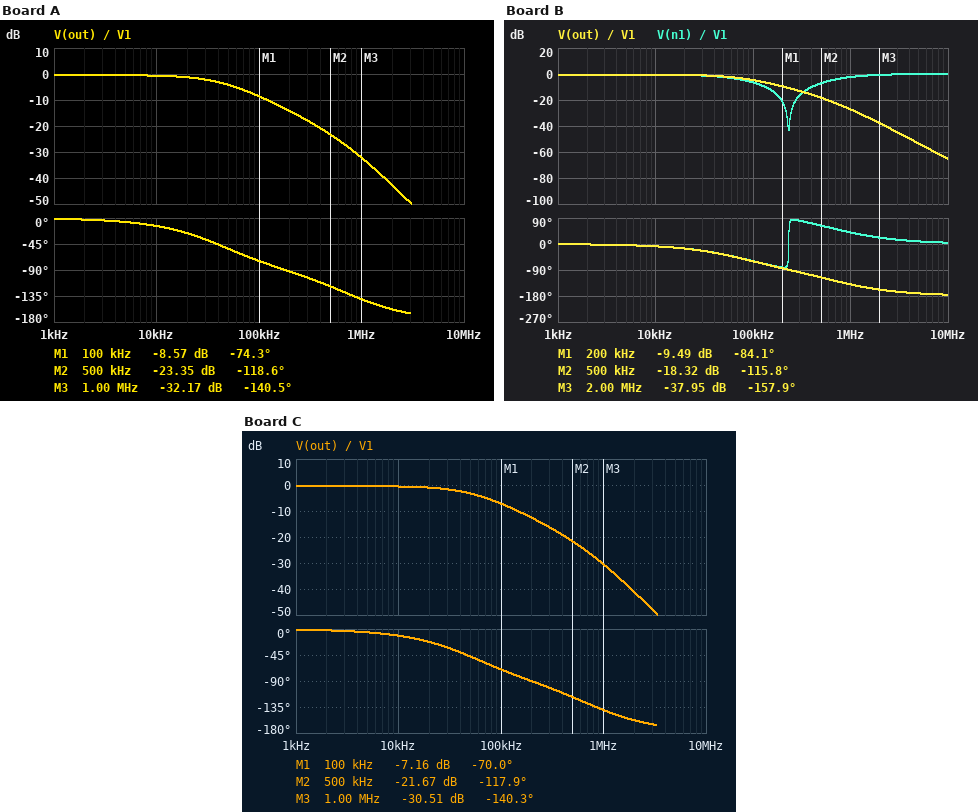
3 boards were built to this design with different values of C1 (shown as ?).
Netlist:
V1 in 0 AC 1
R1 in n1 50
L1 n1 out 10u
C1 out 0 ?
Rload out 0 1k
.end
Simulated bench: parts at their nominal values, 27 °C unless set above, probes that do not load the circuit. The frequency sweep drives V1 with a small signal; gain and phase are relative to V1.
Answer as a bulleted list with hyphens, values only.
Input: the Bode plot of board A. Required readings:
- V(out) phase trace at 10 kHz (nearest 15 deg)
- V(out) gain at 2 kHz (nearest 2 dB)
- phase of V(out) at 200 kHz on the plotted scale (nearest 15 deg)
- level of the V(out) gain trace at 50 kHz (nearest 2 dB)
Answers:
- -15 deg
- 0 dB
- -90 deg
- -4 dB
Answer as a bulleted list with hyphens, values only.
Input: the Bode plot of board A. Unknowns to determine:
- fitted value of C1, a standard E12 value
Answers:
- 82 nF
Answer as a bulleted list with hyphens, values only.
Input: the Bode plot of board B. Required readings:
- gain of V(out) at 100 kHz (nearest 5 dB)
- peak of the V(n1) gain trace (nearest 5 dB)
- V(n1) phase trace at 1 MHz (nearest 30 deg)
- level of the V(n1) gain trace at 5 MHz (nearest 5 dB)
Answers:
- -5 dB
- 0 dB
- 30 deg
- 0 dB
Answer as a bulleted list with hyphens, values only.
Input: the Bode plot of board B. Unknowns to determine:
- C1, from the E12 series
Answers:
- 47 nF
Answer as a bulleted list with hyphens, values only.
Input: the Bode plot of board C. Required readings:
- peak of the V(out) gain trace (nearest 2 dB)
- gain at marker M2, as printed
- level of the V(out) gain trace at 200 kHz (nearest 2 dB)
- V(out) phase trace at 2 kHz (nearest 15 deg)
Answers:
- 0 dB
- -21.67 dB
- -12 dB
- 0 deg
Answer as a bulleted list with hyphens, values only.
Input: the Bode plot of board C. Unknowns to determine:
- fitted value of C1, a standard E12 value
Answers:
- 68 nF
